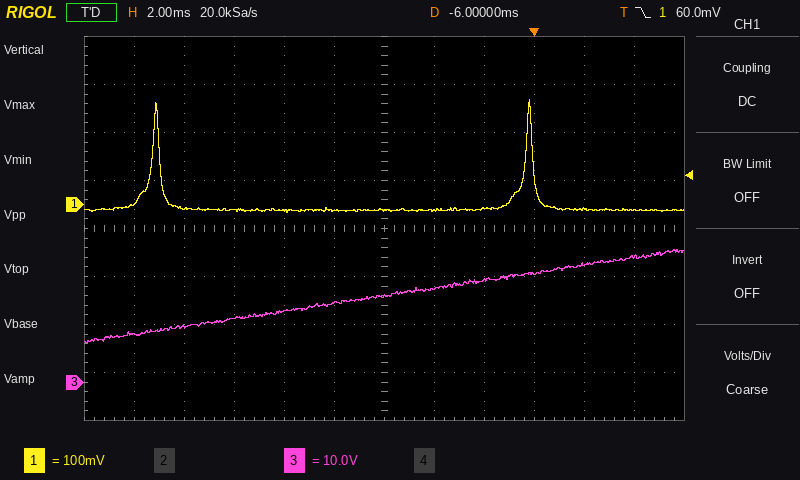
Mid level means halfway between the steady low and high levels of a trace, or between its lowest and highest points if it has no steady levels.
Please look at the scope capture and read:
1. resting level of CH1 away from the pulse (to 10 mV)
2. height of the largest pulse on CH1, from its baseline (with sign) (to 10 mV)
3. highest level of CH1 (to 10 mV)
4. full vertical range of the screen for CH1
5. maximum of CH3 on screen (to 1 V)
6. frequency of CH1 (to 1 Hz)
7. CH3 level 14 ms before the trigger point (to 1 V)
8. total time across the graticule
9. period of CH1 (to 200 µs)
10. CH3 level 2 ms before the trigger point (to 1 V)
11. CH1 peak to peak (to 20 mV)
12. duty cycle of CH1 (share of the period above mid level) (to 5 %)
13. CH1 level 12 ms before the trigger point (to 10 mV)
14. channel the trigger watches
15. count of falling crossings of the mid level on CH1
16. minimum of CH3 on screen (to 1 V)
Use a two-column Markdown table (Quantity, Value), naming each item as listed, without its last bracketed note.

| Quantity | Value |
|---|---|
| resting level of CH1 away from the pulse | -10 mV |
| height of the largest pulse on CH1, from its baseline (with sign) | +230 mV |
| highest level of CH1 | 220 mV |
| full vertical range of the screen for CH1 | 800 mV |
| maximum of CH3 on screen | 28 V |
| frequency of CH1 | 67 Hz |
| CH3 level 14 ms before the trigger point | 12 V |
| total time across the graticule | 24 ms |
| period of CH1 | 15.0 ms |
| CH3 level 2 ms before the trigger point | 21 V |
| CH1 peak to peak | 240 mV |
| duty cycle of CH1 (share of the period above mid level) | 0 % |
| CH1 level 12 ms before the trigger point | -10 mV |
| channel the trigger watches | CH1 |
| count of falling crossings of the mid level on CH1 | 2 |
| minimum of CH3 on screen | 8 V |
